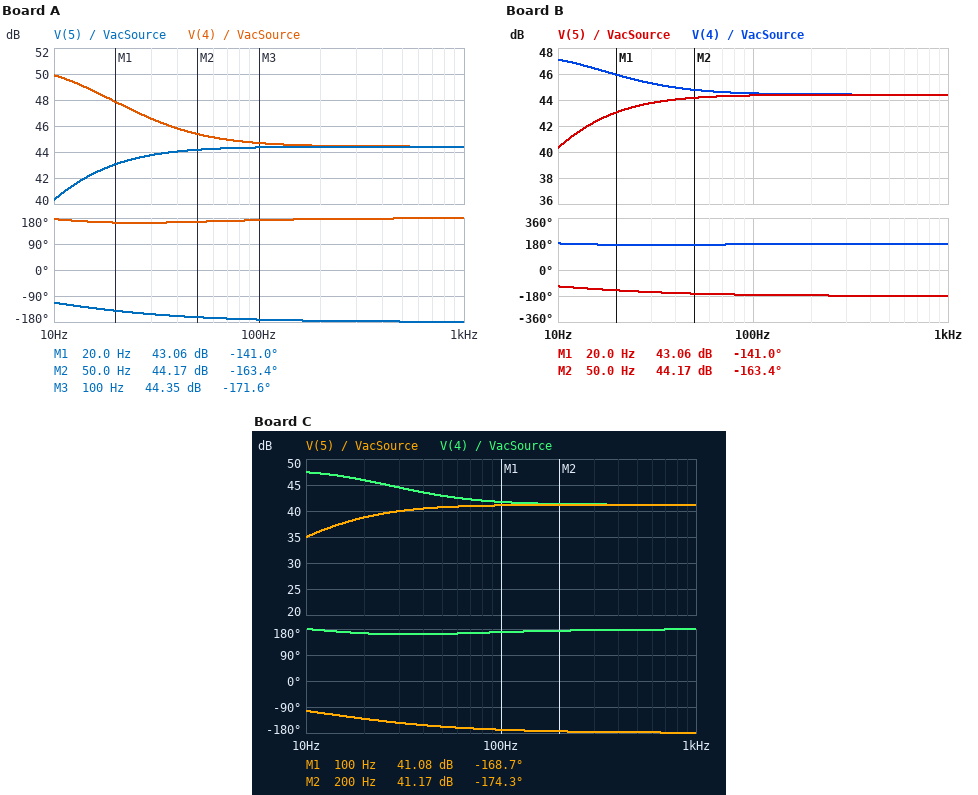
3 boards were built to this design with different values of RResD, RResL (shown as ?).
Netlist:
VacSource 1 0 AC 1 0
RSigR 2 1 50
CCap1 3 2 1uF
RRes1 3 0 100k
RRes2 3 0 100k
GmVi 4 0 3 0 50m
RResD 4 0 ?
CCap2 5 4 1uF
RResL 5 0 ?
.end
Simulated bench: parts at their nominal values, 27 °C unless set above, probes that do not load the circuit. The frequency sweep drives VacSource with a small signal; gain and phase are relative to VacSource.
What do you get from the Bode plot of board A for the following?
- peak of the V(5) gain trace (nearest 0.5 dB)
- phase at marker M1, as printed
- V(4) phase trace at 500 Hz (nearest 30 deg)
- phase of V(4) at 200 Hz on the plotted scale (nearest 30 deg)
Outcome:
44.5 dB
-141.0 deg
180 deg
180 deg
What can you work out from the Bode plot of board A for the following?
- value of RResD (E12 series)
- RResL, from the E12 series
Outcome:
8.2 kΩ
5.6 kΩ
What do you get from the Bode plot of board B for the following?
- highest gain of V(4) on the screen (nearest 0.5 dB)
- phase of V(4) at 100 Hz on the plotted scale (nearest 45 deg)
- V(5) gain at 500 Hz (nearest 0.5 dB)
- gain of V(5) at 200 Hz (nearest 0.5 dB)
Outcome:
47.0 dB
180 deg
44.5 dB
44.5 dB
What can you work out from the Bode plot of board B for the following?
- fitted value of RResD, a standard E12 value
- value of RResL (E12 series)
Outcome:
5.6 kΩ
8.2 kΩ
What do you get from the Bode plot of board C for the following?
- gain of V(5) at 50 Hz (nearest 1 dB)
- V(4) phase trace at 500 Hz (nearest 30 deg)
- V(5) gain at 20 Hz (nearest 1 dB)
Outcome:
41 dB
180 deg
39 dB
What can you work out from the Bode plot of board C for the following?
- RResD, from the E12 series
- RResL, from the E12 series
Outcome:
5.6 kΩ
3.9 kΩ
